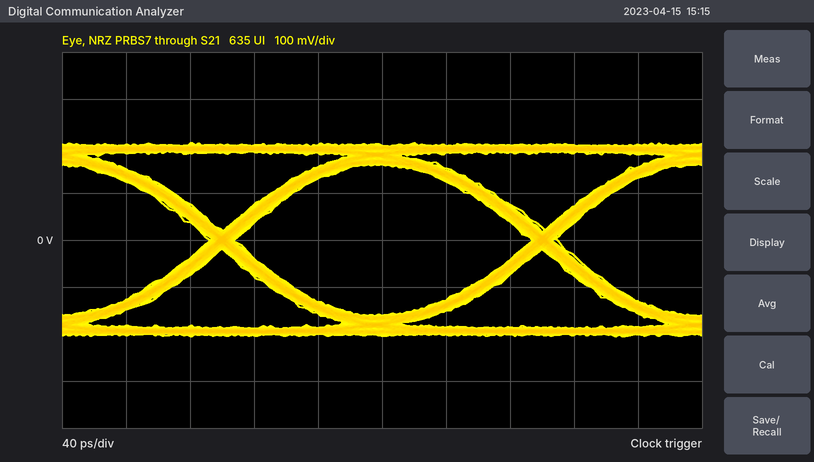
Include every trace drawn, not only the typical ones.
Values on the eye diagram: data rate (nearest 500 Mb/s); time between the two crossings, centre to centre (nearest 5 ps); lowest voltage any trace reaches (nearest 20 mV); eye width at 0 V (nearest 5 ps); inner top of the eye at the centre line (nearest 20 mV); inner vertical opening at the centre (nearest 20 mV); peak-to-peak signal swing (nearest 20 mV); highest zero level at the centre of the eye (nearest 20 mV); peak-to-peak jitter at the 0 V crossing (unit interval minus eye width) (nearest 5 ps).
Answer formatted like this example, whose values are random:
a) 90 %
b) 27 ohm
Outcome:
a) 5.0 Gb/s
b) 200 ps
c) -200 mV
d) 185 ps
e) 160 mV
f) 320 mV
g) 420 mV
h) -160 mV
i) 15 ps
